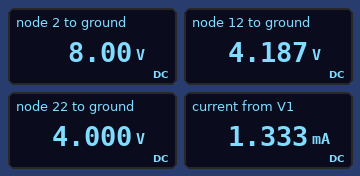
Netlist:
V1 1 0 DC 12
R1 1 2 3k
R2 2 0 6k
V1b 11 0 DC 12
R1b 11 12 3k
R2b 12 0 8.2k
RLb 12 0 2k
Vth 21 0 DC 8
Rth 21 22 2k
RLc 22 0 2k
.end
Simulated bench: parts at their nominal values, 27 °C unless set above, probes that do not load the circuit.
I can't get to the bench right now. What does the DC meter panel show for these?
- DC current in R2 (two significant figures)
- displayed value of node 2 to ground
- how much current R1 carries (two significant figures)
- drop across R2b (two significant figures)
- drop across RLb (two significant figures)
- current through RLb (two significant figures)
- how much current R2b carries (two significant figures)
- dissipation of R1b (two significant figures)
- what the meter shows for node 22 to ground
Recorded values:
1.3 mA
8.00 V
1.3 mA
4.2 V
4.2 V
2.1 mA
510 µA
20 mW
4.000 V
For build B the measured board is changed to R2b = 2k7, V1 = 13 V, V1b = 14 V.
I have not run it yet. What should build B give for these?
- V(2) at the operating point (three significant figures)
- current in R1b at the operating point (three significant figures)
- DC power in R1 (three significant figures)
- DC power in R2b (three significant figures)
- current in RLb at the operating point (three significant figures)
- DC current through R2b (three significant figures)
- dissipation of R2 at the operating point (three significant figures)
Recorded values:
8.67 V
3.37 mA
6.26 mW
5.57 mW
1.94 mA
1.44 mA
12.5 mW
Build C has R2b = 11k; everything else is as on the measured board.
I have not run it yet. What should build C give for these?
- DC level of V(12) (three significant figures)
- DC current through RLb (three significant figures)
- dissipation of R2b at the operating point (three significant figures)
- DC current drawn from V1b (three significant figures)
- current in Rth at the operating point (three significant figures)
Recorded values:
4.33 V
2.16 mA
1.70 mW
2.56 mA
2.00 mA
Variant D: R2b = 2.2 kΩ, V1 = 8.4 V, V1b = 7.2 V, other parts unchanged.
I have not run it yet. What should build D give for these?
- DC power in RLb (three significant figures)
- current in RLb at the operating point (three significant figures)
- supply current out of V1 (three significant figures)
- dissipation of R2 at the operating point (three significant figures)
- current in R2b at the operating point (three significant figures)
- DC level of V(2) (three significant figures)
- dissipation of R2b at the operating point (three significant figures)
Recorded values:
1.74 mW
932 µA
933 µA
5.23 mW
847 µA
5.60 V
1.58 mW
